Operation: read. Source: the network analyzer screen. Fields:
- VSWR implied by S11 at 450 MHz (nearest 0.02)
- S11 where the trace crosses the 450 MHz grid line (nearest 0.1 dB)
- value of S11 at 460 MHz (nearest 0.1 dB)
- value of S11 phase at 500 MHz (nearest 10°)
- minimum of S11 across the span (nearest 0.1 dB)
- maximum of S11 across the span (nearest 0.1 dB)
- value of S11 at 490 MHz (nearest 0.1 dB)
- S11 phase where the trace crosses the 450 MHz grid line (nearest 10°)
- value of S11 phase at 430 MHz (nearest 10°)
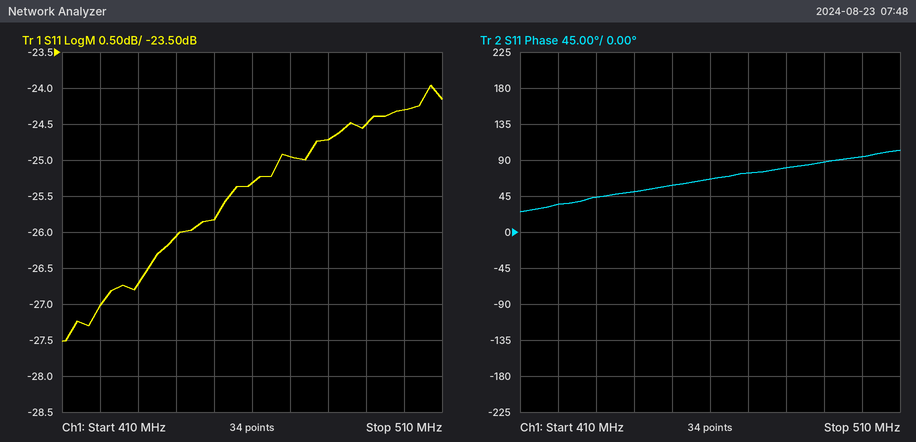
1.10
-25.8 dB
-25.3 dB
90°
-27.5 dB
-24.0 dB
-24.5 dB
60°
40°
